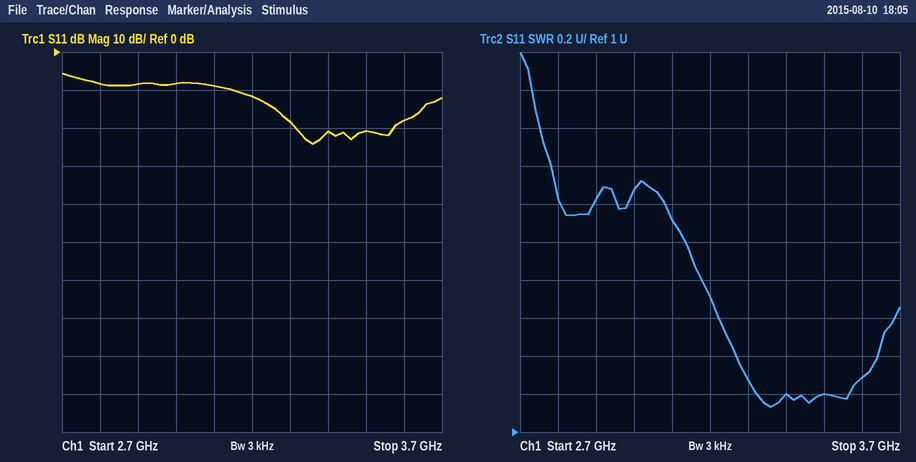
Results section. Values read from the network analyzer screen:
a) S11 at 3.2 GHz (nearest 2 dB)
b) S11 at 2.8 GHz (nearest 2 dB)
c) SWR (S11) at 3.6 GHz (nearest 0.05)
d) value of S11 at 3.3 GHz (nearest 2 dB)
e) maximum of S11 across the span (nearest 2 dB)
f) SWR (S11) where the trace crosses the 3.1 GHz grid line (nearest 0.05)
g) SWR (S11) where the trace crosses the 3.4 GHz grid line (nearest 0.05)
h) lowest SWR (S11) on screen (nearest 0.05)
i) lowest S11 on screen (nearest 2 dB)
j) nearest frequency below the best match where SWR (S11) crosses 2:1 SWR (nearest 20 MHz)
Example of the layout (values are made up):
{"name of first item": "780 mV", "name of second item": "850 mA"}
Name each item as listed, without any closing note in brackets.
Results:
{"S11 at 3.2 GHz": "-12 dB", "S11 at 2.8 GHz": "-8 dB", "SWR (S11) at 3.6 GHz": "1.30", "value of S11 at 3.3 GHz": "-18 dB", "maximum of S11 across the span": "-6 dB", "SWR (S11) where the trace crosses the 3.1 GHz grid line": "2.10", "SWR (S11) where the trace crosses the 3.4 GHz grid line": "1.20", "lowest SWR (S11) on screen": "1.15", "lowest S11 on screen": "-24 dB", "nearest frequency below the best match where SWR (S11) crosses 2:1 SWR": "3.14 GHz"}
